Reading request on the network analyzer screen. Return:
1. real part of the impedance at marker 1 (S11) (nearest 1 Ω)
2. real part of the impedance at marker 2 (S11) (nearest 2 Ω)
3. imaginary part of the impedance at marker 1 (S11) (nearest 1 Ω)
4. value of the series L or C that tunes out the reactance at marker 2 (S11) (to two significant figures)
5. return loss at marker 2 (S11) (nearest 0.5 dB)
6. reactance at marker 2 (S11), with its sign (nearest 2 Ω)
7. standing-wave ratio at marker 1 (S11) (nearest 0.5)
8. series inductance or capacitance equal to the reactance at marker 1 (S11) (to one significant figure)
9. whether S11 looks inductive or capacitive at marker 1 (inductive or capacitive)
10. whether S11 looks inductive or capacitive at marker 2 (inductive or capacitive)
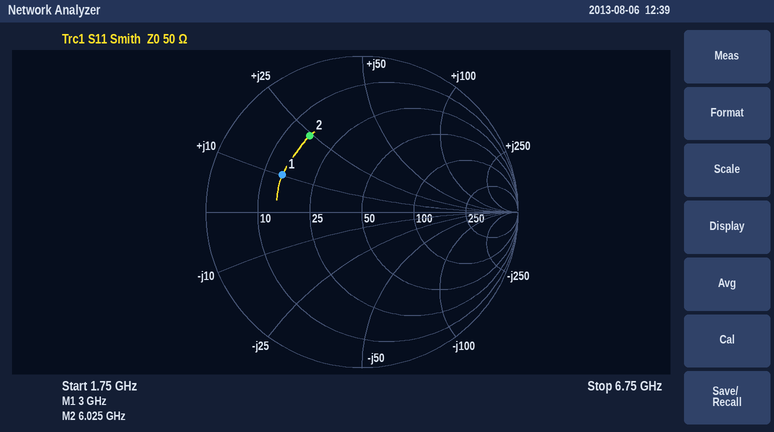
15 Ω
16 Ω
+10 Ω
1.1 pF
4.5 dB
+24 Ω
3.5
500 pH
inductive
inductive
